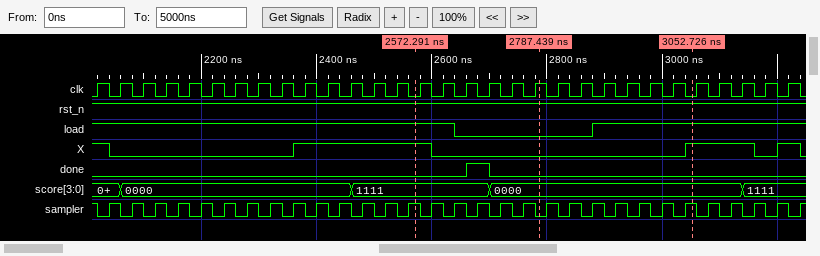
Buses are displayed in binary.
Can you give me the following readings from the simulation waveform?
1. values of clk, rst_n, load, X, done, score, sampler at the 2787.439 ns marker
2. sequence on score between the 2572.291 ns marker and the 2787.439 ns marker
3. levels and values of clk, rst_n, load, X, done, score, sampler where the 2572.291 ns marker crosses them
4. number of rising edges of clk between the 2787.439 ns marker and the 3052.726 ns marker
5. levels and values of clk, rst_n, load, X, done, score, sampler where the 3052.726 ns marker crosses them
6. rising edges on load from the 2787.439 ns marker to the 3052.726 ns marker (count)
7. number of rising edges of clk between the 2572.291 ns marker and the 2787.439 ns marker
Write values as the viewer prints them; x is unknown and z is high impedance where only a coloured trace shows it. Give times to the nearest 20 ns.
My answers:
clk=1, rst_n=1, load=0, X=0, done=0, score=0000, sampler=0
1111, 0000
clk=0, rst_n=1, load=1, X=1, done=0, score=1111, sampler=1
6
clk=0, rst_n=1, load=1, X=1, done=0, score=0000, sampler=1
1
6
